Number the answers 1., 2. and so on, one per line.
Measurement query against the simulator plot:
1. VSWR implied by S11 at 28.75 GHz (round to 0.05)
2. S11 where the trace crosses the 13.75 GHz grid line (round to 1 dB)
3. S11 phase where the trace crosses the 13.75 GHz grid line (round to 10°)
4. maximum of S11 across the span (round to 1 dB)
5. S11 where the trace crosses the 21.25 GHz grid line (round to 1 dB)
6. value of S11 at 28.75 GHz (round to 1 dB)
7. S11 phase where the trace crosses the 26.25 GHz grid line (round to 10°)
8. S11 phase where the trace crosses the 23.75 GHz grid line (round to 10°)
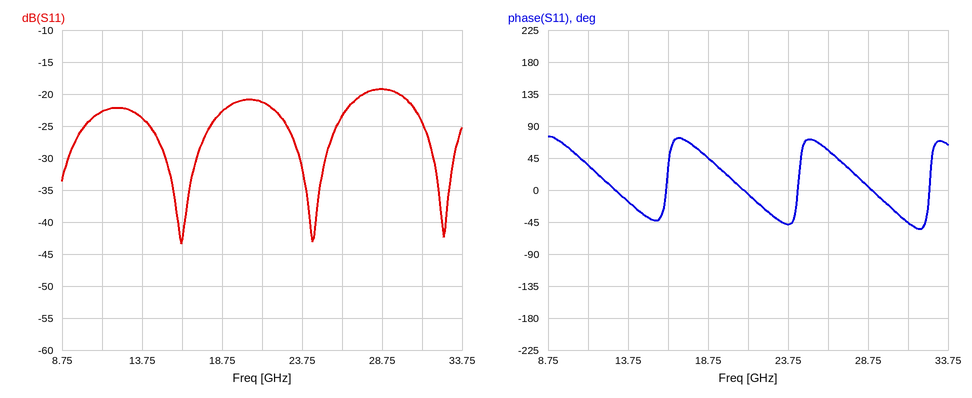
1. 1.25
2. -24 dB
3. -20°
4. -19 dB
5. -21 dB
6. -19 dB
7. 60°
8. -50°
